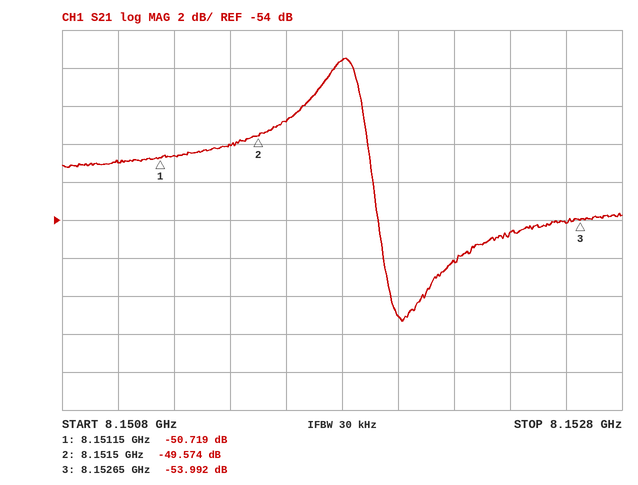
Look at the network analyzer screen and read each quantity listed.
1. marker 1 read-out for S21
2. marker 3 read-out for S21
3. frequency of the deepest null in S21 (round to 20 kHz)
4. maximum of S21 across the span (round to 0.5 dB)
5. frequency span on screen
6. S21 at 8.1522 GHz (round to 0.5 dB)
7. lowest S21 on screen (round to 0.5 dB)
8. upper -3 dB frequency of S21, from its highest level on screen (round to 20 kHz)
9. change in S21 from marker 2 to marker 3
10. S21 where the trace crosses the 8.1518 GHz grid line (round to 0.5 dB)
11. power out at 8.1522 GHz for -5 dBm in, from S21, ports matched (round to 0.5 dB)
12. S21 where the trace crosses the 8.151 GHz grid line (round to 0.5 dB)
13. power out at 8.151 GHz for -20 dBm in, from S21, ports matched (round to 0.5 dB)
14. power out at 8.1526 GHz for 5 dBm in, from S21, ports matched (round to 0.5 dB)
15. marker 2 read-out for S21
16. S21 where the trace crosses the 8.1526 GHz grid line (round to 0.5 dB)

-50.719 dB
-53.992 dB
8.15202 GHz
-45.5 dB
2 MHz
-56.0 dB
-59.5 dB
8.15188 GHz
-4.418 dB
-45.5 dB
-61.0 dBm
-51.0 dB
-71.0 dBm
-49.0 dBm
-49.574 dB
-54.0 dB
